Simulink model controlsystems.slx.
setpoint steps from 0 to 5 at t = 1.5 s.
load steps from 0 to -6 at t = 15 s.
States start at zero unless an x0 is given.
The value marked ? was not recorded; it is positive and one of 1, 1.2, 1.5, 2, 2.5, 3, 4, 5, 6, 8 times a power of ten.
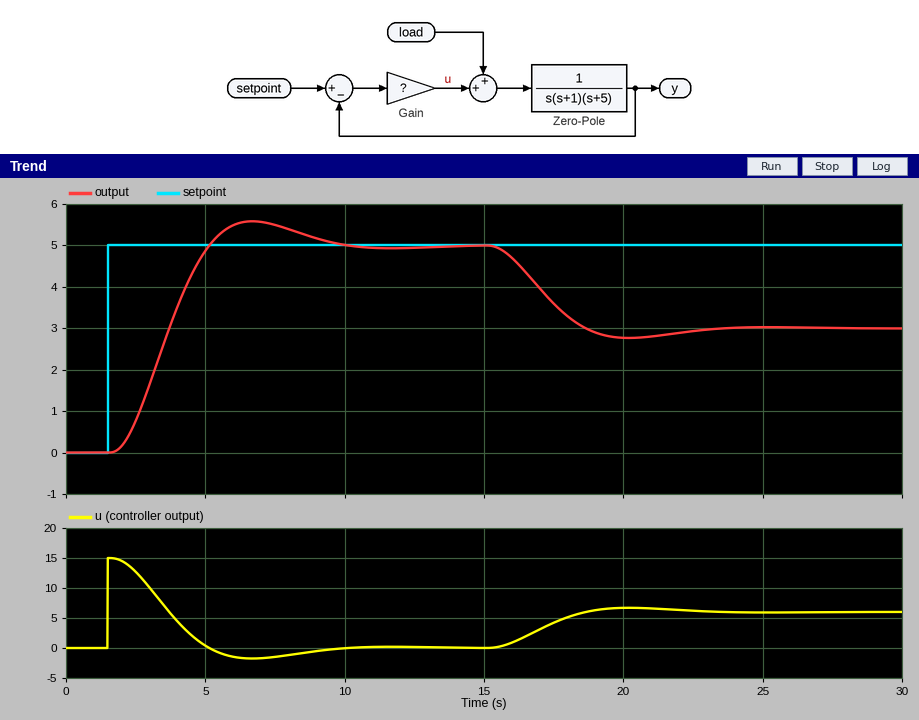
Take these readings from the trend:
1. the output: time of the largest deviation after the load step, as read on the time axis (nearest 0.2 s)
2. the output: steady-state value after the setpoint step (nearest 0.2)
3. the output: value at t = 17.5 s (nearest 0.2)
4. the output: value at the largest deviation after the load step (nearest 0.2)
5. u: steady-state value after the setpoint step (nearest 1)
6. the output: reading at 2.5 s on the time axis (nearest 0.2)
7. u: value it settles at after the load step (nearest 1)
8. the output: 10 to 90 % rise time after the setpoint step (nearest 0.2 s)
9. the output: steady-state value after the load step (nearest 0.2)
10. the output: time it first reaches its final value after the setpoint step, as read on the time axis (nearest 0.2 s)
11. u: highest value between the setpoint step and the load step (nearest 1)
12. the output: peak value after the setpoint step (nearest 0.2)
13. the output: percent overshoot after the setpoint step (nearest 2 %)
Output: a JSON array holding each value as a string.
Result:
["20.2 s", "5.0", "3.6", "2.8", "0", "0.8", "6", "2.4 s", "3.0", "5.2 s", "15", "5.6", "12 %"]
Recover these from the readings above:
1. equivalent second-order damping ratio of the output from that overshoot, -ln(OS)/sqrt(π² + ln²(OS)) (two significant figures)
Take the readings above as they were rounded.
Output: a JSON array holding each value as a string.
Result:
["0.56"]
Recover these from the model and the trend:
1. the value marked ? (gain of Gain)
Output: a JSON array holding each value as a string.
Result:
["3"]
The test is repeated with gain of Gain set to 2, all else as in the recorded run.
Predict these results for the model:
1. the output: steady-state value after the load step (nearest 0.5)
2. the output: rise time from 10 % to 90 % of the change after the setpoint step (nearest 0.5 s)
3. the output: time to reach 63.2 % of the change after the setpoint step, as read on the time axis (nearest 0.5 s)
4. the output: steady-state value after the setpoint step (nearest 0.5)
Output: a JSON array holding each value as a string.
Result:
["2.0", "3.5 s", "4.5 s", "5.0"]
